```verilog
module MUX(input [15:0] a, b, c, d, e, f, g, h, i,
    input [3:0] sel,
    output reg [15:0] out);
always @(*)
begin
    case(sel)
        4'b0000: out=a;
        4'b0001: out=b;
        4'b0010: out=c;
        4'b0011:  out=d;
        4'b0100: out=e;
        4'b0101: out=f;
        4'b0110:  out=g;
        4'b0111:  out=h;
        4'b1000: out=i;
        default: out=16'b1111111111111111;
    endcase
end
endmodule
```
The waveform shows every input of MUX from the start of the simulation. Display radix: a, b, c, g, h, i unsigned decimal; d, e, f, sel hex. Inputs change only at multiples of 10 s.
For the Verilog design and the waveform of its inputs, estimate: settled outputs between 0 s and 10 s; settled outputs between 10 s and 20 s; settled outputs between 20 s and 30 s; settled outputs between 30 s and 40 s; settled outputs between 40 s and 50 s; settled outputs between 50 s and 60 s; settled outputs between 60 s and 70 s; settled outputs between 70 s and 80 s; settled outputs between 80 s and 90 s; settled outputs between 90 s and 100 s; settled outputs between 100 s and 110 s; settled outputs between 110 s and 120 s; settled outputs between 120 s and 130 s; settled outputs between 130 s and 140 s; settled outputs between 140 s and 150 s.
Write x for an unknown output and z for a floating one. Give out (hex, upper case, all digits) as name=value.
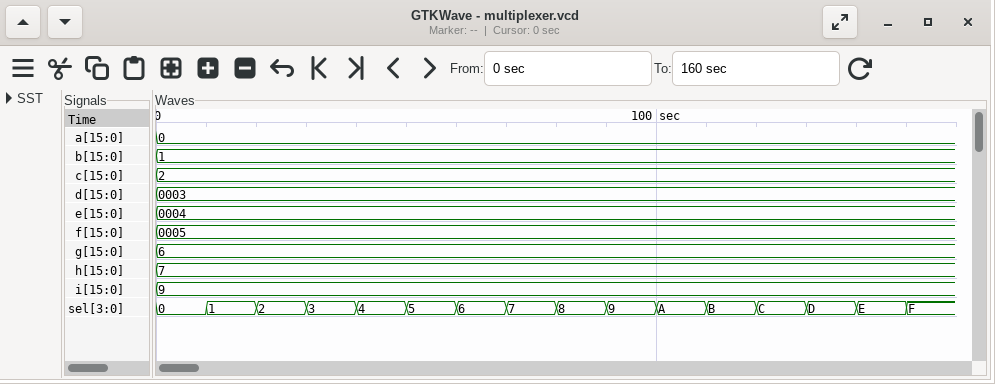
out=0000
out=0001
out=0002
out=0003
out=0004
out=0005
out=0006
out=0007
out=0009
out=FFFF
out=FFFF
out=FFFF
out=FFFF
out=FFFF
out=FFFF
